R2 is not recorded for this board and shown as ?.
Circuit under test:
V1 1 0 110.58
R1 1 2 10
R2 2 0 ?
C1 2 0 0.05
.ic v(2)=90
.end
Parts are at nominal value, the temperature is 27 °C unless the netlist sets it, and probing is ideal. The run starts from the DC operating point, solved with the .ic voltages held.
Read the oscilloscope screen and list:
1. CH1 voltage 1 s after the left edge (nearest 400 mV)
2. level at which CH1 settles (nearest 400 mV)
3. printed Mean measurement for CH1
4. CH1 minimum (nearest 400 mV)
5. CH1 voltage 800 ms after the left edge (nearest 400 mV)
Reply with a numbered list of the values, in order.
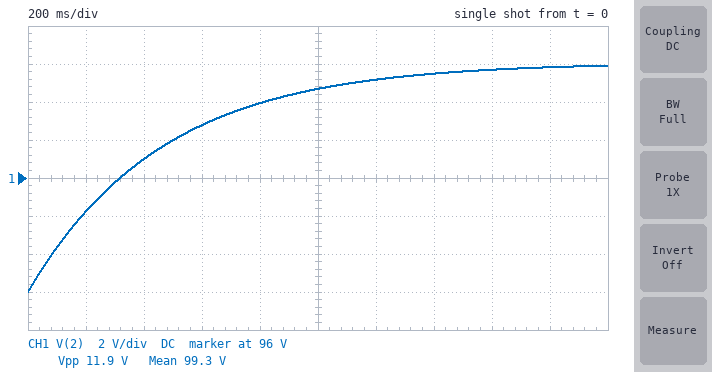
1. 100.8 V
2. 102.0 V
3. 99.3 V
4. 90.0 V
5. 100.0 V
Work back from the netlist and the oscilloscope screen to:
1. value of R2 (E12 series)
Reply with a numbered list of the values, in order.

1. 120 Ω
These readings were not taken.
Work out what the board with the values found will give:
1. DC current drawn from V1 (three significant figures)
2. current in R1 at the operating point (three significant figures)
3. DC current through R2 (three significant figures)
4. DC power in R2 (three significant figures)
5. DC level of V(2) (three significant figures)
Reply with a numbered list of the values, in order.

1. 851 mA
2. 851 mA
3. 851 mA
4. 86.8 W
5. 102 V
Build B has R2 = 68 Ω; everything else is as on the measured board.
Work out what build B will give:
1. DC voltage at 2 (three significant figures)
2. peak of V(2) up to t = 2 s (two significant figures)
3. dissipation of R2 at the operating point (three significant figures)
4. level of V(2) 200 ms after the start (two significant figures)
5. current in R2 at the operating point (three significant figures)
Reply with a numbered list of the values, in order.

1. 96.4 V
2. 96 V
3. 137 W
4. 92 V
5. 1.42 A
